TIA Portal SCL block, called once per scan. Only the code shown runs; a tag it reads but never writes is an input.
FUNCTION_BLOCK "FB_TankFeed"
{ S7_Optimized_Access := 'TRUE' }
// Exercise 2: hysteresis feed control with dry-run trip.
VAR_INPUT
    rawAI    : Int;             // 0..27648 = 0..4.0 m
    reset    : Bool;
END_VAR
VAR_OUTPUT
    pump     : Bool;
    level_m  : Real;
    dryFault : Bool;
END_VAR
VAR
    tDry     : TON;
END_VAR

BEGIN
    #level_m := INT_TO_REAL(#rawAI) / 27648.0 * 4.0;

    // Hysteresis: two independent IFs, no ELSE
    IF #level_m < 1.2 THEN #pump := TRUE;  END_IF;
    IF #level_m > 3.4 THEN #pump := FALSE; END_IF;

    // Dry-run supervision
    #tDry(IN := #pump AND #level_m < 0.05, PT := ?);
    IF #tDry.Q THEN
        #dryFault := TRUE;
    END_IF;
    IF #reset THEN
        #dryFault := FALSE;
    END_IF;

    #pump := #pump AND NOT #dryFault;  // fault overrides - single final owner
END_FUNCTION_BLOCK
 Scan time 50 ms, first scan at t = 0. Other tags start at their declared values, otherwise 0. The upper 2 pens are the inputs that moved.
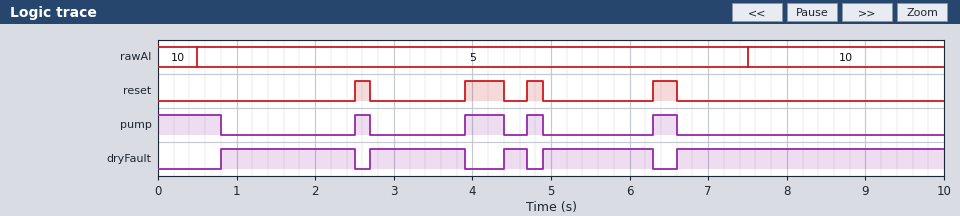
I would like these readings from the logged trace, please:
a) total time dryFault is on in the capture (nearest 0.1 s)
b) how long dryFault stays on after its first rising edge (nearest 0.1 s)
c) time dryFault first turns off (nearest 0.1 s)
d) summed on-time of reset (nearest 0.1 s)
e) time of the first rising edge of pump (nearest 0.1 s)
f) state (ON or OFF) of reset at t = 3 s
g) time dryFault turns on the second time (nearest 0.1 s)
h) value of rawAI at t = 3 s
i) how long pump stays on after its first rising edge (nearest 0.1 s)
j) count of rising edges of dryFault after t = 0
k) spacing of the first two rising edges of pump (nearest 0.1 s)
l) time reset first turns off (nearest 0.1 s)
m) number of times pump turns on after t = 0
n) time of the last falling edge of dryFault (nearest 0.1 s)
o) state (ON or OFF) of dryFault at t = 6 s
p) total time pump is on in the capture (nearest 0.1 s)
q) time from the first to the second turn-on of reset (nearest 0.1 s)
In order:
8.0 s
1.7 s
2.5 s
1.2 s
2.5 s
OFF
2.7 s
5
0.2 s
5
1.4 s
2.7 s
4
6.3 s
ON
2.0 s
1.4 s
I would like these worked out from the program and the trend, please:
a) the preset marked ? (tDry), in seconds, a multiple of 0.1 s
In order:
0.8 s
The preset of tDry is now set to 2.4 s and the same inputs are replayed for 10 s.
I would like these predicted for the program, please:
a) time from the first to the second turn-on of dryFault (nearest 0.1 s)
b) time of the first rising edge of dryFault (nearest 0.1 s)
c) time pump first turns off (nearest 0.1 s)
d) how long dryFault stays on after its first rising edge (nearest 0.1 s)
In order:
0.3 s
2.4 s
2.4 s
0.1 s
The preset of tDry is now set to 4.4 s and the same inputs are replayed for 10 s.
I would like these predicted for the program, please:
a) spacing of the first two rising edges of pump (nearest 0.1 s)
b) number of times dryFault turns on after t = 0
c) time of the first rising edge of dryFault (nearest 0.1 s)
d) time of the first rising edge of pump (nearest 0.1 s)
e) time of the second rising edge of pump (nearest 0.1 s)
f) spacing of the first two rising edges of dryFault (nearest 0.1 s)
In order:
1.6 s
3
4.4 s
4.7 s
6.3 s
0.5 s
